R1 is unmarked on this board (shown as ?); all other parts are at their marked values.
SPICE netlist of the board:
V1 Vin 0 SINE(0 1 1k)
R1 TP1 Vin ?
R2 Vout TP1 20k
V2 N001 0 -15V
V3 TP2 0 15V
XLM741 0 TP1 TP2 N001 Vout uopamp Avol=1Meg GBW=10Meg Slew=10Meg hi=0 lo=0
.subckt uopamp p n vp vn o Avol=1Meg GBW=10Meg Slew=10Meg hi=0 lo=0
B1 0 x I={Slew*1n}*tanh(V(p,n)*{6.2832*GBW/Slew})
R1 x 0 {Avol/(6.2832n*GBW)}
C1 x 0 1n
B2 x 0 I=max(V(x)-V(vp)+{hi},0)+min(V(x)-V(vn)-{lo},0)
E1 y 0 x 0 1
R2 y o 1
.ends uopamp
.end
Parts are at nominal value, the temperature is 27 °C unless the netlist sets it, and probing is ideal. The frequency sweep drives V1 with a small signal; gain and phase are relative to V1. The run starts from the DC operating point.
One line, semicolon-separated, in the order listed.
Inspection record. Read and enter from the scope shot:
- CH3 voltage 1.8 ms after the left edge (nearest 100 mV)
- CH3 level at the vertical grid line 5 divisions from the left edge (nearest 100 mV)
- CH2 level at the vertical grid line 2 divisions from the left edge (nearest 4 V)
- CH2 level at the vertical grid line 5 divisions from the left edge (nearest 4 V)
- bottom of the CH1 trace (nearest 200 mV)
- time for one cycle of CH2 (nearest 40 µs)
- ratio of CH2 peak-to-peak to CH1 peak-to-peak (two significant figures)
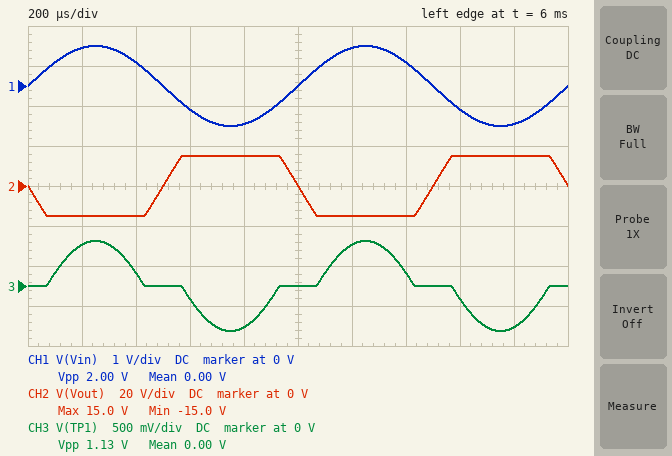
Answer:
-500 mV; 0 V; -16 V; 0 V; -1.0 V; 1.00 ms; 15
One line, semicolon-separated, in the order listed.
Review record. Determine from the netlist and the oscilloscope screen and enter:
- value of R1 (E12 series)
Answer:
560 Ω
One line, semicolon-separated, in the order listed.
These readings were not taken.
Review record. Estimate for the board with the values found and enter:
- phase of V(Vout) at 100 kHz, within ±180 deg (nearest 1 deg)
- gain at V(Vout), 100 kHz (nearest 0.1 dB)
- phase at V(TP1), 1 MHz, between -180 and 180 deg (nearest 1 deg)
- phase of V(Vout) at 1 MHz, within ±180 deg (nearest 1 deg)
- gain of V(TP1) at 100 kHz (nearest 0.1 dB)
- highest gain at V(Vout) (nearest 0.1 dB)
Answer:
160 deg; 30.5 dB; 15 deg; 105 deg; -9.5 dB; 31.1 dB
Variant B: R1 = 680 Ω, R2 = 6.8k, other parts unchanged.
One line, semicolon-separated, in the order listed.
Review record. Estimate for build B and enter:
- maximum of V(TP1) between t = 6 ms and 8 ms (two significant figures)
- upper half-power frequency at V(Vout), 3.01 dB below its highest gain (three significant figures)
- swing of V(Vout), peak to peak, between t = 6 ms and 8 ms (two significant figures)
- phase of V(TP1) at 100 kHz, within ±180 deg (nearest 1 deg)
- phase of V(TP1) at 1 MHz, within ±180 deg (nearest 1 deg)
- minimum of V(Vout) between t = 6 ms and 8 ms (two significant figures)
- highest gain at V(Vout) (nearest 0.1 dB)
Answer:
1.0 mV; 909 kHz; 20 V; 84 deg; 42 deg; -10 V; 20.0 dB
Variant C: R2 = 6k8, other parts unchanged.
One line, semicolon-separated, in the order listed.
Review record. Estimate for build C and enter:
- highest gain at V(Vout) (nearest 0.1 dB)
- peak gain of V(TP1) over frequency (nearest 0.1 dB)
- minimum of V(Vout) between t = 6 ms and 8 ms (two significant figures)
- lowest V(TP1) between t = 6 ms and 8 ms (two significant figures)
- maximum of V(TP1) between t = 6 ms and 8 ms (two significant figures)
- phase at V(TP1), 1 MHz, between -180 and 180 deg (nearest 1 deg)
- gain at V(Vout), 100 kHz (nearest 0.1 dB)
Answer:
21.7 dB; -0.7 dB; -12 V; -1.2 mV; 1.2 mV; 37 deg; 21.6 dB
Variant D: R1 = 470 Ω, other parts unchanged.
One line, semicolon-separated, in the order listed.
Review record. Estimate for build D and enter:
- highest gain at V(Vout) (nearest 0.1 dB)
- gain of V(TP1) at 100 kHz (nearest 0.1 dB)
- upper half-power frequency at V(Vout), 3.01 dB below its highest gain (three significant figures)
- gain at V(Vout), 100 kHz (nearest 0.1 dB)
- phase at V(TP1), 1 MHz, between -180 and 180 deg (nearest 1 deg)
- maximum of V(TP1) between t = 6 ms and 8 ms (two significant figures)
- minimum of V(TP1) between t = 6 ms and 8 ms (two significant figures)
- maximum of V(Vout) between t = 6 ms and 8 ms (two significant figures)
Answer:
32.6 dB; -8.2 dB; 230 kHz; 31.8 dB; 13 deg; 630 mV; -630 mV; 15 V
